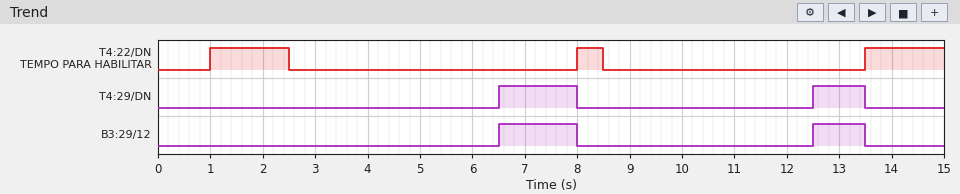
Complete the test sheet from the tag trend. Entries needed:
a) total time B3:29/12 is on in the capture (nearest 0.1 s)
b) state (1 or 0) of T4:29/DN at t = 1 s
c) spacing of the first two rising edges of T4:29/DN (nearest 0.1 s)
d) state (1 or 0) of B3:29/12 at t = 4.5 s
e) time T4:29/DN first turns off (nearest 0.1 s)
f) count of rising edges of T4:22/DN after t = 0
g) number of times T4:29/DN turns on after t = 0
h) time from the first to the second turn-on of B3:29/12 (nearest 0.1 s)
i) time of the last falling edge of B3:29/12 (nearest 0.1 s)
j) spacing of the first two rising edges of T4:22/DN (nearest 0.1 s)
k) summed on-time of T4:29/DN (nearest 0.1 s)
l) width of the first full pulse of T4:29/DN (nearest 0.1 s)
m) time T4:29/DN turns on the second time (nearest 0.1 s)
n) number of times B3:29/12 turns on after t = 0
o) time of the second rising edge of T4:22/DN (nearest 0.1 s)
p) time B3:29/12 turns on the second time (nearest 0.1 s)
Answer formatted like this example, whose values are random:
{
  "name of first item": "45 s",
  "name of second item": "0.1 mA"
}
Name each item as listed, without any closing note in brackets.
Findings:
{
  "total time B3:29/12 is on in the capture": "2.5 s",
  "state (1 or 0) of T4:29/DN at t = 1 s": "0",
  "spacing of the first two rising edges of T4:29/DN": "6.0 s",
  "state (1 or 0) of B3:29/12 at t = 4.5 s": "0",
  "time T4:29/DN first turns off": "8.0 s",
  "count of rising edges of T4:22/DN after t = 0": "3",
  "number of times T4:29/DN turns on after t = 0": "2",
  "time from the first to the second turn-on of B3:29/12": "6.0 s",
  "time of the last falling edge of B3:29/12": "13.5 s",
  "spacing of the first two rising edges of T4:22/DN": "7.0 s",
  "summed on-time of T4:29/DN": "2.5 s",
  "width of the first full pulse of T4:29/DN": "1.5 s",
  "time T4:29/DN turns on the second time": "12.5 s",
  "number of times B3:29/12 turns on after t = 0": "2",
  "time of the second rising edge of T4:22/DN": "8.0 s",
  "time B3:29/12 turns on the second time": "12.5 s"
}
